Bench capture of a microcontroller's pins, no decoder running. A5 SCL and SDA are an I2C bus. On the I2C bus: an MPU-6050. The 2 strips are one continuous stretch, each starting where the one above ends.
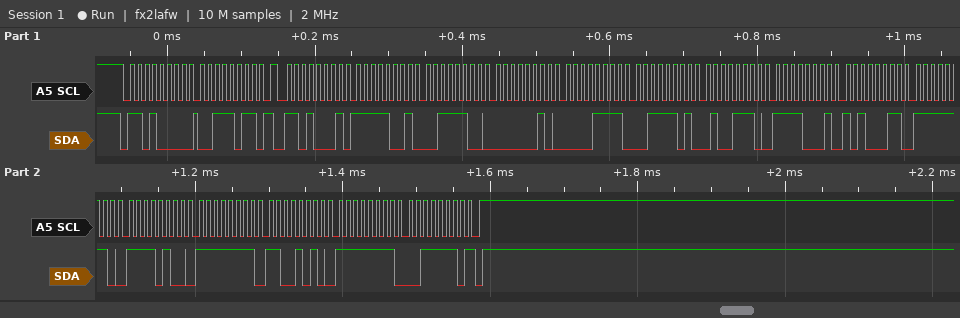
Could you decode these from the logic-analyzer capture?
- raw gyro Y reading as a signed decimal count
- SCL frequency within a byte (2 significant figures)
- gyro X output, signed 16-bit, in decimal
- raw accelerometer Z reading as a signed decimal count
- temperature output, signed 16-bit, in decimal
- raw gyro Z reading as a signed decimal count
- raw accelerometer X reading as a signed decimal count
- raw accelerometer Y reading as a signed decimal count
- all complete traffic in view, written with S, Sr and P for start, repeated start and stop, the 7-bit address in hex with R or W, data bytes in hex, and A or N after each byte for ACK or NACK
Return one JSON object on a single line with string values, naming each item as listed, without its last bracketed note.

{"raw gyro Y reading as a signed decimal count": "-54", "SCL frequency within a byte": "100 kHz", "gyro X output, signed 16-bit, in decimal": "-268", "raw accelerometer Z reading as a signed decimal count": "15694", "temperature output, signed 16-bit, in decimal": "-3677", "raw gyro Z reading as a signed decimal count": "-194", "raw accelerometer X reading as a signed decimal count": "-1732", "raw accelerometer Y reading as a signed decimal count": "527", "all complete traffic in view, written with S, Sr and P for start, repeated start and stop, the 7-bit address in hex with R or W, data bytes in hex, and A or N after each byte for ACK or NACK": "S 68W A 3B A Sr 68R A F9 A 3C A 02 A 0F A 3D A 4E A F1 A A3 A FE A F4 A FF A CA A FF A 3E N P"}
